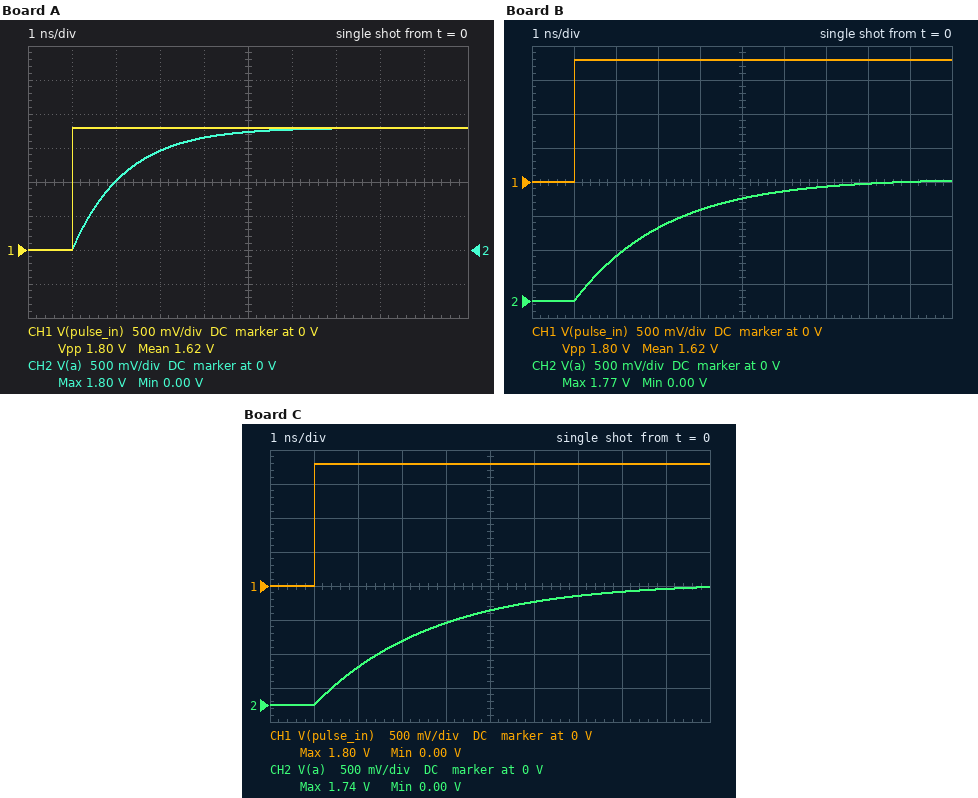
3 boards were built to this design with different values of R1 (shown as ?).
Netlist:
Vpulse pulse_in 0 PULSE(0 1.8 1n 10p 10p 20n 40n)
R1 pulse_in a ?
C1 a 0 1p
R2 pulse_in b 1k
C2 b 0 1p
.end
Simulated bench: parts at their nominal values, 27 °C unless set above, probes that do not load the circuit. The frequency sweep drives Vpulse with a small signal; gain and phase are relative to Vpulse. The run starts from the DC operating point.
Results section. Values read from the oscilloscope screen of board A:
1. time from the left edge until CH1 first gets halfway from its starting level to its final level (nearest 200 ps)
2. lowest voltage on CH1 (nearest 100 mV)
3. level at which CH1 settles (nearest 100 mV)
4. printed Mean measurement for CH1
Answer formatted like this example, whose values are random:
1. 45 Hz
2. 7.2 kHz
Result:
1. 1.0 ns
2. 0 V
3. 1.8 V
4. 1.62 V
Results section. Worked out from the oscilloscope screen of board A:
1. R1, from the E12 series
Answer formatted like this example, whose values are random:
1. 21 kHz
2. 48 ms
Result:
1. 1.2 kΩ
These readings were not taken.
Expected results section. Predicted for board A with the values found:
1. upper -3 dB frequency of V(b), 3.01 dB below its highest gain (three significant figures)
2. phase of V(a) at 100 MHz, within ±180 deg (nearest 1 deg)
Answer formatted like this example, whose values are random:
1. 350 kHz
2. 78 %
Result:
1. 159 MHz
2. -37 deg
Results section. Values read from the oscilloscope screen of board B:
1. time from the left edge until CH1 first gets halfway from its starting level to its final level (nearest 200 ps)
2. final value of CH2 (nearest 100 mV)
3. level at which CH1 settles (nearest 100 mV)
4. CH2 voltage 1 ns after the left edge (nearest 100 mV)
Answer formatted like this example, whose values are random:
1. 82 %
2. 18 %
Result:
1. 1.0 ns
2. 1.8 V
3. 1.8 V
4. 0 V
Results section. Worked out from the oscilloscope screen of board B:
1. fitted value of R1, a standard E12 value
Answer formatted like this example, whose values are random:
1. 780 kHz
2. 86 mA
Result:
1. 2.2 kΩ
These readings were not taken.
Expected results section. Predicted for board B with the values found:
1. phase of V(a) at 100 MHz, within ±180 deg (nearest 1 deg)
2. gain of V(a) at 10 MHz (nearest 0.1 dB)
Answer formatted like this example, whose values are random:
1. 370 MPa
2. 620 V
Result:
1. -54 deg
2. -0.1 dB
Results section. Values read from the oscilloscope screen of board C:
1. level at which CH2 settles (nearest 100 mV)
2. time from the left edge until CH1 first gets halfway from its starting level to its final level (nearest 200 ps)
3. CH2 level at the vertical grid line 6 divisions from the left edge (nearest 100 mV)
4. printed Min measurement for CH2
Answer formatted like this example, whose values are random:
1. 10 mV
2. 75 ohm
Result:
1. 1.7 V
2. 1.0 ns
3. 1.5 V
4. 0.00 V
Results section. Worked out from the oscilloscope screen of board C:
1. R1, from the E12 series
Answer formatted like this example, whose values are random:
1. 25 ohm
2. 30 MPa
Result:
1. 2.7 kΩ
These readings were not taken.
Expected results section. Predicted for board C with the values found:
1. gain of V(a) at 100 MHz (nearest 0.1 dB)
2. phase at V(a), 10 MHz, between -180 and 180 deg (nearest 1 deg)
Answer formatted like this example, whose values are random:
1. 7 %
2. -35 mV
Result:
1. -5.9 dB
2. -10 deg
